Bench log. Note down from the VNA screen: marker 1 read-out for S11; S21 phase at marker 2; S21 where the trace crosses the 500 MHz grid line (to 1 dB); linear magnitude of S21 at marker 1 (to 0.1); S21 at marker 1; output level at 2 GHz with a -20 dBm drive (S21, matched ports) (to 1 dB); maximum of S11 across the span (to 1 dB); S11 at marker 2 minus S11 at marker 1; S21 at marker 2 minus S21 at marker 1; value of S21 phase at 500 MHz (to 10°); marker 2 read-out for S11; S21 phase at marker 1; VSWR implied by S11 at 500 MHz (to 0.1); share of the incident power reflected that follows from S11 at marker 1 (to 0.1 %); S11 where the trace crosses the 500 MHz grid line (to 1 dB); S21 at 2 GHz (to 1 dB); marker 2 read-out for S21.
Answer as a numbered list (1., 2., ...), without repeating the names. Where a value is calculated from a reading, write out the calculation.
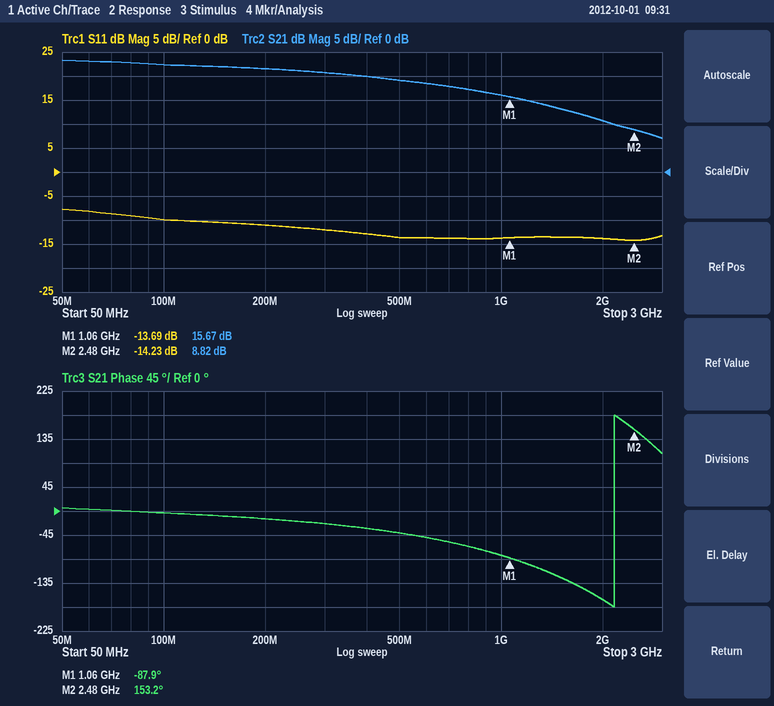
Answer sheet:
1. -13.69 dB
2. 153.2°
3. 19 dB
4. 10^(15.67/20) ≈ 6.1
5. 15.67 dB
6. -20 dBm + (11 dB) = -9 dBm
7. -8 dB
8. -14.23 − (-13.69) = -0.54 dB
9. 8.82 − (15.67) = -6.85 dB
10. -40°
11. -14.23 dB
12. -87.9°
13. |Γ| = 10^(-14/20) = 0.1995; VSWR = (1 + 0.1995)/(1 − 0.1995) ≈ 1.5
14. 10^(-13.69/10) ≈ 4.3 %
15. -14 dB
16. 11 dB
17. 8.82 dB
